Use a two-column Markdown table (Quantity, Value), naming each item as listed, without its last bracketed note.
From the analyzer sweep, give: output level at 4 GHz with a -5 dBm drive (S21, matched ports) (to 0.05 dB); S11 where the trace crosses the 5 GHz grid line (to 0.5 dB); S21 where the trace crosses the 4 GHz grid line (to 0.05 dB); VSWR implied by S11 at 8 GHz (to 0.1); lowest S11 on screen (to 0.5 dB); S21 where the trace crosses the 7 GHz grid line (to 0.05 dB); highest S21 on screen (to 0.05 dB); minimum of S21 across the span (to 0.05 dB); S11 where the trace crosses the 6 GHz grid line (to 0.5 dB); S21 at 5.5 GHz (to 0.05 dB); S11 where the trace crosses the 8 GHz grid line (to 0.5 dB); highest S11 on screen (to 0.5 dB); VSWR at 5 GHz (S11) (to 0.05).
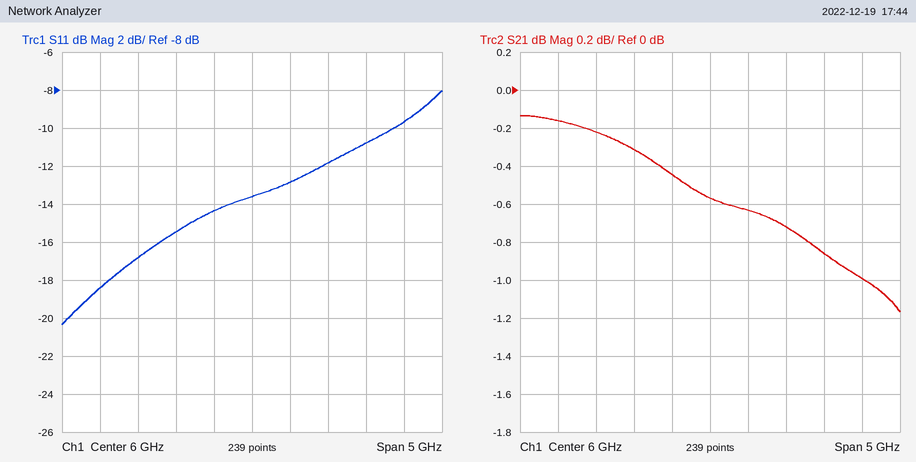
| Quantity | Value |
|---|---|
| output level at 4 GHz with a -5 dBm drive (S21, matched ports) | -5.15 dBm |
| S11 where the trace crosses the 5 GHz grid line | -15.5 dB |
| S21 where the trace crosses the 4 GHz grid line | -0.15 dB |
| VSWR implied by S11 at 8 GHz | 2.0 |
| lowest S11 on screen | -20.5 dB |
| S21 where the trace crosses the 7 GHz grid line | -0.70 dB |
| highest S21 on screen | -0.15 dB |
| minimum of S21 across the span | -1.15 dB |
| S11 where the trace crosses the 6 GHz grid line | -13.5 dB |
| S21 at 5.5 GHz | -0.45 dB |
| S11 where the trace crosses the 8 GHz grid line | -9.5 dB |
| highest S11 on screen | -8.0 dB |
| VSWR at 5 GHz (S11) | 1.40 |
